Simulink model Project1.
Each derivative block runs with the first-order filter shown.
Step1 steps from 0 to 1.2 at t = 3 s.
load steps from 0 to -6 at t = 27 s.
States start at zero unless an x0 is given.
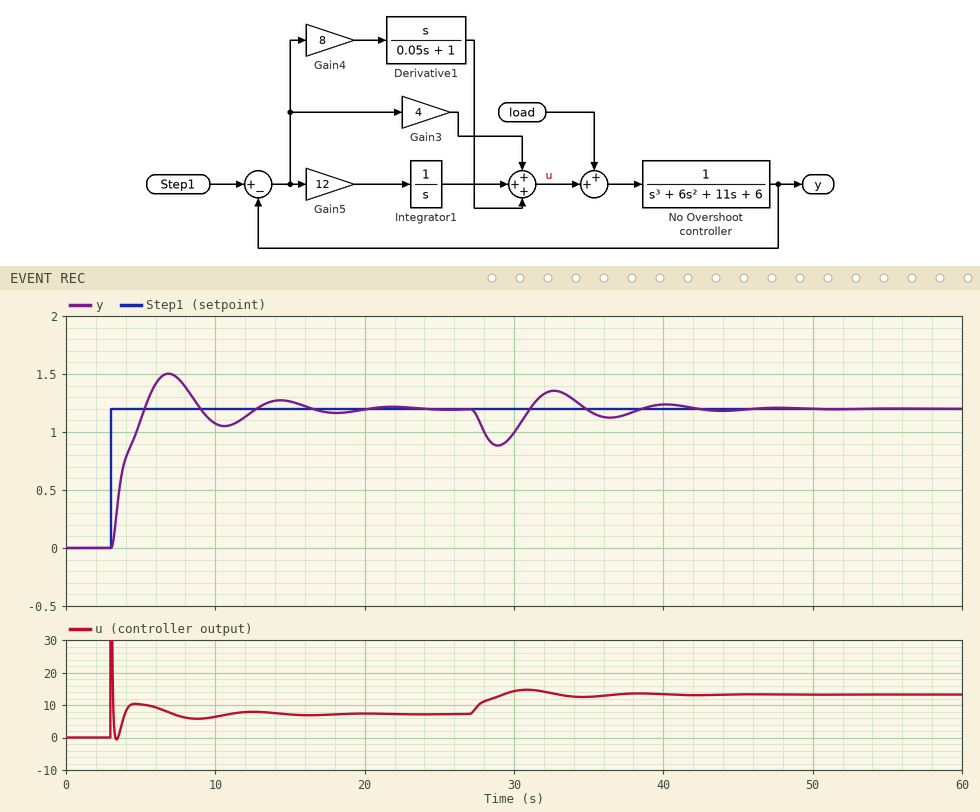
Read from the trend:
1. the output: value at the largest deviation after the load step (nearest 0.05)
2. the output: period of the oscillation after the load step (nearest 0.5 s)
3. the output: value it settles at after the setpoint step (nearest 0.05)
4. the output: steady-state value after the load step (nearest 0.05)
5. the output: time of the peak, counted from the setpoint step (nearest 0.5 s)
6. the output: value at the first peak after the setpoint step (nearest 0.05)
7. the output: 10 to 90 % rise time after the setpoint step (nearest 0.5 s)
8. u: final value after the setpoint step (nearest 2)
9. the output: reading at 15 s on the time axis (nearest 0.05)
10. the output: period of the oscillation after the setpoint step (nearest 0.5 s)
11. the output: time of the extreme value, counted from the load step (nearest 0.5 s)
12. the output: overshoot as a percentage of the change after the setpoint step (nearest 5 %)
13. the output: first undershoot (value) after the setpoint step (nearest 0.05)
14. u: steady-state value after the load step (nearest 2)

0.90
7.5 s
1.20
1.20
4.0 s
1.50
1.5 s
8
1.25
7.5 s
2.0 s
25 %
1.05
14
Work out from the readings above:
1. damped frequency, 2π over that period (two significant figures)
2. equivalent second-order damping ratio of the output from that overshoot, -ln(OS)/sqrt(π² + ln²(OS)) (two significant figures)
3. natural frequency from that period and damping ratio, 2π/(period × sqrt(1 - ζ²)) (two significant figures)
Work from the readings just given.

0.84 rad/s
0.40
0.91 rad/s
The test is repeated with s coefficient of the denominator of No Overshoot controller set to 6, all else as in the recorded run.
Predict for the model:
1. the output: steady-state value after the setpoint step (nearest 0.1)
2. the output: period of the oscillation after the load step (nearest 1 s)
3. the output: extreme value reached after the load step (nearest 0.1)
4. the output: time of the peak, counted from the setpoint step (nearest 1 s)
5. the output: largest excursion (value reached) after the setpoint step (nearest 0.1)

1.2
6 s
0.8
3 s
1.4
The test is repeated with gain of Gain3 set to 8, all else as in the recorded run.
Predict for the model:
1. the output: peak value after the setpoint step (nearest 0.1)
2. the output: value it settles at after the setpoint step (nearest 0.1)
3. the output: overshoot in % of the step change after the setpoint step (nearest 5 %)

1.4
1.2
15 %
